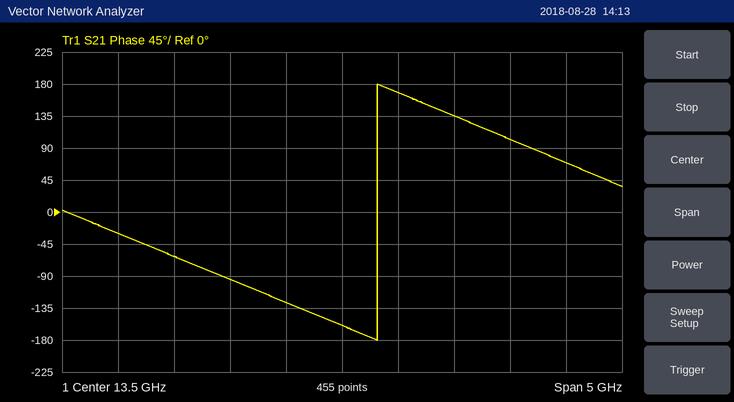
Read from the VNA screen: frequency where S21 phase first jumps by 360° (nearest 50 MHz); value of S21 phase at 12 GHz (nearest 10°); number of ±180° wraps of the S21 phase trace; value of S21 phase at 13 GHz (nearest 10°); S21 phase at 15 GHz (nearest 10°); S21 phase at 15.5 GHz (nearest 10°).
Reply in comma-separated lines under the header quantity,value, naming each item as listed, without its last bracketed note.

quantity,value
frequency where S21 phase first jumps by 360°,13.80 GHz
value of S21 phase at 12 GHz,-60°
number of ±180° wraps of the S21 phase trace,1
value of S21 phase at 13 GHz,-130°
S21 phase at 15 GHz,100°
S21 phase at 15.5 GHz,70°
